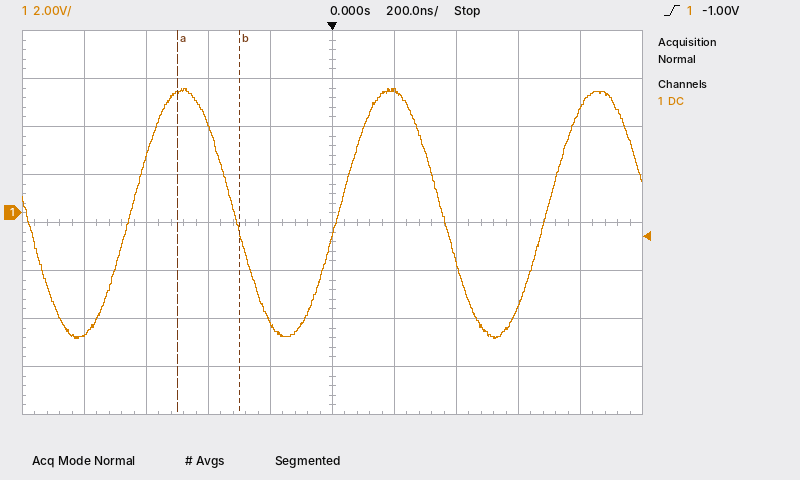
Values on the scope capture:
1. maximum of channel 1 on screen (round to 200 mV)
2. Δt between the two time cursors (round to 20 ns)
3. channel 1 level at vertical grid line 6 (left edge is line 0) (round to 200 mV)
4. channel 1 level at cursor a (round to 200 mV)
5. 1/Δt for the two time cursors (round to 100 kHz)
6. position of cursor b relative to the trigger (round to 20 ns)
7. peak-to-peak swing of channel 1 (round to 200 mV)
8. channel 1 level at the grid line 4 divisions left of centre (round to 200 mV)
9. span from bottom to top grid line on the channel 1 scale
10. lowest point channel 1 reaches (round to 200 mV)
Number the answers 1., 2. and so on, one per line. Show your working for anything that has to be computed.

1. 5.2 V
2. 200 ns
3. 5.0 V
4. 5.0 V
5. 1 / 200 ns ≈ 5.0 MHz
6. -300 ns
7. 5.2 V − (-5.2 V) = 10.4 V
8. -5.0 V
9. 16 V
10. -5.2 V
